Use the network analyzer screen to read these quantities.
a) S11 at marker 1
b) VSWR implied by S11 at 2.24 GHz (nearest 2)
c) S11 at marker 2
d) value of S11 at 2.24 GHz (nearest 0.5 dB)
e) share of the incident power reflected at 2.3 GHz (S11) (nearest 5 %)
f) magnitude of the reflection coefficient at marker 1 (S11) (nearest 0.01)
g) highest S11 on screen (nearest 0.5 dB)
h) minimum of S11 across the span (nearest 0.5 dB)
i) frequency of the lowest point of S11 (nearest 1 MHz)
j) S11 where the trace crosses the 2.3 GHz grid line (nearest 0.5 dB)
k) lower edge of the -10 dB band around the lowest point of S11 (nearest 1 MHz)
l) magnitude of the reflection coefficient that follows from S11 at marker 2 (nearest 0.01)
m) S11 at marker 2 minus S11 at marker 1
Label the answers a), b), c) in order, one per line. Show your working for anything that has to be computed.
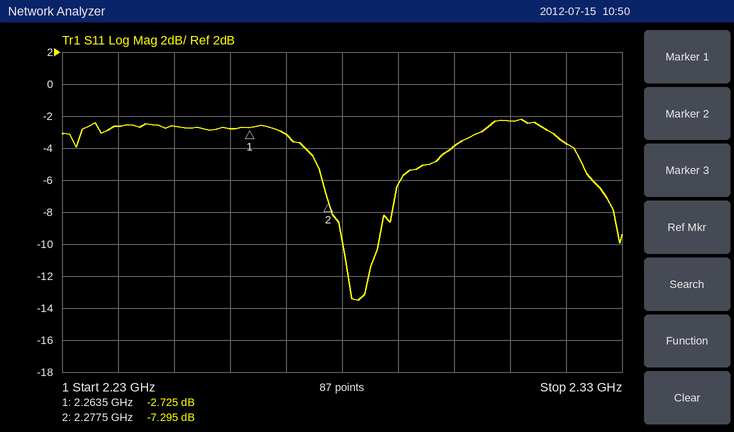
a) -2.725 dB
b) |Γ| = 10^(-2.5/20) = 0.7499; VSWR = (1 + 0.7499)/(1 − 0.7499) ≈ 7.00, so 6 to the nearest 2
c) -7.295 dB
d) -2.5 dB
e) 10^(-4/10) ≈ 40 %
f) 10^(-2.725/20) ≈ 0.73
g) -2.0 dB
h) -13.5 dB
i) 2.283 GHz
j) -4.0 dB
k) 2.280 GHz
l) 10^(-7.295/20) ≈ 0.43
m) -7.295 − (-2.725) = -4.570 dB
